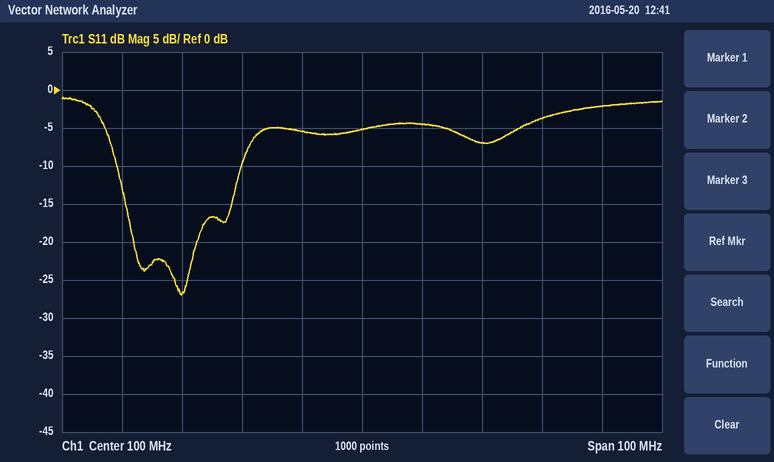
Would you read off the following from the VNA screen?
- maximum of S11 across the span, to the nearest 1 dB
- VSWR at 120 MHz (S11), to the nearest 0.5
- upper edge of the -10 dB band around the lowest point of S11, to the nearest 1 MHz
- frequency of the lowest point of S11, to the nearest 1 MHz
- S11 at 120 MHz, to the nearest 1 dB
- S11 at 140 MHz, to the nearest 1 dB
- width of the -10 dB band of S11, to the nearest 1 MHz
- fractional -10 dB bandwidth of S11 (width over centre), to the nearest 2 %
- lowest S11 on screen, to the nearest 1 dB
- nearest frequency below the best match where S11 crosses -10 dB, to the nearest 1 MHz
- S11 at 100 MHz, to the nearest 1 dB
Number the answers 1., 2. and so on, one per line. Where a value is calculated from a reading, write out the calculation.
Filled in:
1. -1 dB
2. |Γ| = 10^(-7/20) = 0.4467; VSWR = (1 + 0.4467)/(1 − 0.4467) ≈ 2.61, so 2.5 to the nearest 0.5
3. 80 MHz
4. 70 MHz
5. -7 dB
6. -2 dB
7. 80 MHz − 59 MHz = 21 MHz
8. 21 MHz / 69.5 MHz ≈ 30 %
9. -27 dB
10. 59 MHz
11. -5 dB
